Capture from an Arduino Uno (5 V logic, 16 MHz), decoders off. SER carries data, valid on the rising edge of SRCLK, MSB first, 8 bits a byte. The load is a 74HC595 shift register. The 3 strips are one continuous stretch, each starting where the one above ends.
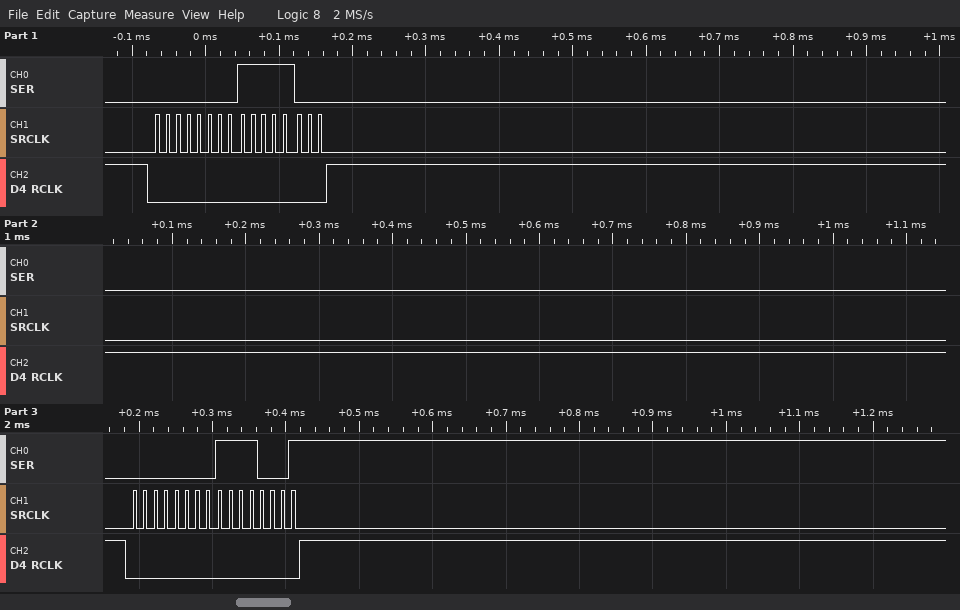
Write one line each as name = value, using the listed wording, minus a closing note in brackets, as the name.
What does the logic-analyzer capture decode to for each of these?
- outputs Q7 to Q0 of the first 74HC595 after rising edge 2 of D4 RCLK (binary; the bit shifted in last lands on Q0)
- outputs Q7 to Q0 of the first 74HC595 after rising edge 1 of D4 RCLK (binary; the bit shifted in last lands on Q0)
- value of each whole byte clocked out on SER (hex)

outputs Q7 to Q0 of the first 74HC595 after rising edge 2 of D4 RCLK = 11110001
outputs Q7 to Q0 of the first 74HC595 after rising edge 1 of D4 RCLK = 11111000
value of each whole byte clocked out on SER = 00 F8 00 F1
